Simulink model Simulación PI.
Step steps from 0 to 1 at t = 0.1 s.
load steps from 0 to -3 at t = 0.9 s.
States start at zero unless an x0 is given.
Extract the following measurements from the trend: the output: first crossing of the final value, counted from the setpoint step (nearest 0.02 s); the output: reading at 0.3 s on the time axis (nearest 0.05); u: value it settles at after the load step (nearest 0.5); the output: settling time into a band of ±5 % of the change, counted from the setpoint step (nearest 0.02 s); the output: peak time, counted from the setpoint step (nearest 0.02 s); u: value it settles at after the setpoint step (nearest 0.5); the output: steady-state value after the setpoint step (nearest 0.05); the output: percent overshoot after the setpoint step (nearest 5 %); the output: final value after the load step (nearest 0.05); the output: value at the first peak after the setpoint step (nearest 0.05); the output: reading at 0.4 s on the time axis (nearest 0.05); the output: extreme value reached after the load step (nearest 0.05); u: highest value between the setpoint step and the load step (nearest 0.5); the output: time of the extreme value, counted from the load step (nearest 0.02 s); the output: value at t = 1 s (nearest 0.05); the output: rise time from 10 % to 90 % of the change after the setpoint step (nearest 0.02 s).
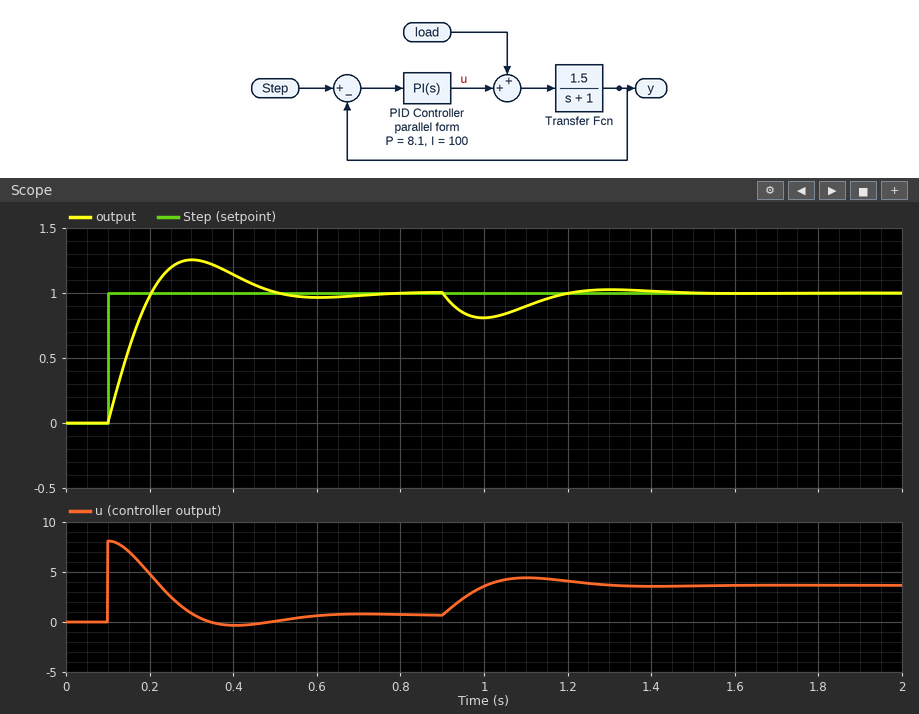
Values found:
0.10 s
1.25
3.5
0.36 s
0.20 s
0.5
1.00
25 %
1.00
1.25
1.15
0.80
8.0
0.10 s
0.80
0.08 s
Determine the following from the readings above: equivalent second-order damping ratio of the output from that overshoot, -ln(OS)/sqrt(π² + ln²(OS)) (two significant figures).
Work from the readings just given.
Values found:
0.40
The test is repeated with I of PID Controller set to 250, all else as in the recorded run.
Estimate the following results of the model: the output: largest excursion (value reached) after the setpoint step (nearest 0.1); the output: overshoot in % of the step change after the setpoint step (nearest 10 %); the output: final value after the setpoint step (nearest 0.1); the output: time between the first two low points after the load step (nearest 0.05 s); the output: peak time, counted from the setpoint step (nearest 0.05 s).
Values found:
1.4
40 %
1.0
0.35 s
0.15 s
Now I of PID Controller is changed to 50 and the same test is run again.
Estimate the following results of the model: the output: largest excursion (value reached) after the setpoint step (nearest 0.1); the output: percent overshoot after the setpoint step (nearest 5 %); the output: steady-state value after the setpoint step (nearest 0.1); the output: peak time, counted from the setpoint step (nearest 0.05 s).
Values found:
1.2
15 %
1.0
0.25 s
